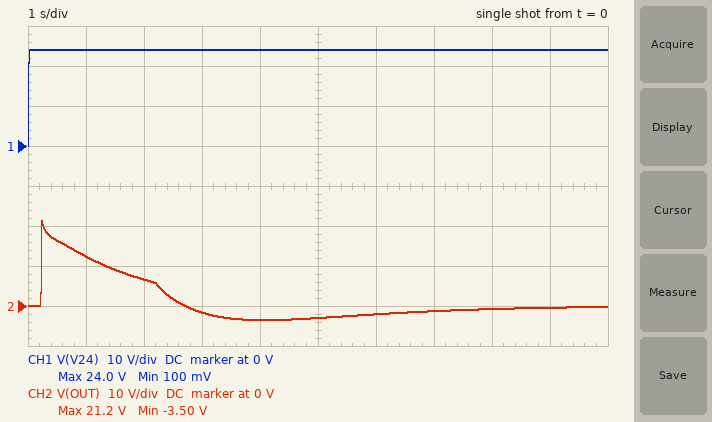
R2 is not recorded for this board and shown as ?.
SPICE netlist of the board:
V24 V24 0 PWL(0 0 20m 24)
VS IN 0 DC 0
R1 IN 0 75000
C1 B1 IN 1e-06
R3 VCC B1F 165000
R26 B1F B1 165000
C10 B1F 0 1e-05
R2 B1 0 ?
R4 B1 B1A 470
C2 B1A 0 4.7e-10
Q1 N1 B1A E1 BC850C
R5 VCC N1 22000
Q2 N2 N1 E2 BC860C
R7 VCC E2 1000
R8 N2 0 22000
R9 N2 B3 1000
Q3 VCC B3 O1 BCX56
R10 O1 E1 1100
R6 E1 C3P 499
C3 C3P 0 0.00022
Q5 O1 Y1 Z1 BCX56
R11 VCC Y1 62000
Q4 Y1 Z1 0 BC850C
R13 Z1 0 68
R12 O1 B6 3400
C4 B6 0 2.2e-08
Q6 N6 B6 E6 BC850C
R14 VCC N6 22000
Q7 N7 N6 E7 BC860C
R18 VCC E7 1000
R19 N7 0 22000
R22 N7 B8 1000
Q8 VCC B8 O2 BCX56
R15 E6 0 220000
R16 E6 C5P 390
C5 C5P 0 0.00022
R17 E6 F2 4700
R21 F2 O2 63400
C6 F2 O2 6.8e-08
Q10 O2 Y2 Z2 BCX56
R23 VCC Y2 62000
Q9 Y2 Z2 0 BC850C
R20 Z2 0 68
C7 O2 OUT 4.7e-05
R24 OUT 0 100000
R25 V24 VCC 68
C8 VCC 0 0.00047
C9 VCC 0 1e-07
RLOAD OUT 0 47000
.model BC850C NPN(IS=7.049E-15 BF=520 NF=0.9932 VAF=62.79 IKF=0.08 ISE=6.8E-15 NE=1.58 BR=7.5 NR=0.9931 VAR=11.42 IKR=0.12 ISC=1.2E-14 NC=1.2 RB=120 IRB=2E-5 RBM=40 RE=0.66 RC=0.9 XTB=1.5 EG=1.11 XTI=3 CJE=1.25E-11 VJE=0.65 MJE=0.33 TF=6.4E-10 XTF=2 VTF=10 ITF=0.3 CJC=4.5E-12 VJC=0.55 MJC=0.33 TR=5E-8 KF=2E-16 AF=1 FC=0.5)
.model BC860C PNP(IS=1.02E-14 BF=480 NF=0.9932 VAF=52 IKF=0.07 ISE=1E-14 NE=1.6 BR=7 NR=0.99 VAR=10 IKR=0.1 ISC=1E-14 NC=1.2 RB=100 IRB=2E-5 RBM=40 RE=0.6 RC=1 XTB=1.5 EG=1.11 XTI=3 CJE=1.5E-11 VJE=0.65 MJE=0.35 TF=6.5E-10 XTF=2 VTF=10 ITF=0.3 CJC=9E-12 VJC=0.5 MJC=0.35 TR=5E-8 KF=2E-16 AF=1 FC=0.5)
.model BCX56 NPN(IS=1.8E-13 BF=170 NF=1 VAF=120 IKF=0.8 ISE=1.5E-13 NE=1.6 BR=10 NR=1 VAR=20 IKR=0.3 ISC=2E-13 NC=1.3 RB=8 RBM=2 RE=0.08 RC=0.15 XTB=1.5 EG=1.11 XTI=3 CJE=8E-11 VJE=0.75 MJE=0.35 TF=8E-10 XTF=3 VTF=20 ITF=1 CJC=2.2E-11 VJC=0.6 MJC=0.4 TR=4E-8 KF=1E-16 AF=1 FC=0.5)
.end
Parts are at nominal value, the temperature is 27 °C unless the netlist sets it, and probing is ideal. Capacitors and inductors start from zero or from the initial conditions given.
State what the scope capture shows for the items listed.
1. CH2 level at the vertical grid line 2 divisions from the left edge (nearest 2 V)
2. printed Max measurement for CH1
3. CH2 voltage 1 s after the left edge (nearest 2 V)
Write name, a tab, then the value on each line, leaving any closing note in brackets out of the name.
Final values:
CH2 level at the vertical grid line 2 divisions from the left edge	6 V
printed Max measurement for CH1	24.0 V
CH2 voltage 1 s after the left edge	12 V
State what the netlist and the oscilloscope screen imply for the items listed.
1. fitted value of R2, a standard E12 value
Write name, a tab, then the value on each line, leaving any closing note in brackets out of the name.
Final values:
fitted value of R2, a standard E12 value	220 kΩ
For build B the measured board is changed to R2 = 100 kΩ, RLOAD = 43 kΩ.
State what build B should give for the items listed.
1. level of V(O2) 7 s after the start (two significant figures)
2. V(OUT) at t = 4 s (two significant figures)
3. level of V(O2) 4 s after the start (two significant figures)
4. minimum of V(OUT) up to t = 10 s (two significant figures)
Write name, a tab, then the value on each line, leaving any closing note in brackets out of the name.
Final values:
level of V(O2) 7 s after the start	2.9 V
V(OUT) at t = 4 s	-3.1 V
level of V(O2) 4 s after the start	4.0 V
minimum of V(OUT) up to t = 10 s	-3.8 V
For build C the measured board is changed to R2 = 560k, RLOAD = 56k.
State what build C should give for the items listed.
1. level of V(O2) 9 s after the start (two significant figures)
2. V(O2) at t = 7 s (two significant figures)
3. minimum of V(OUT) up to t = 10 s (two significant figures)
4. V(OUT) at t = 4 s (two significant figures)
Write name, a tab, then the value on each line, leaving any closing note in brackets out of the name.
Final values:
level of V(O2) 9 s after the start	13 V
V(O2) at t = 7 s	14 V
minimum of V(OUT) up to t = 10 s	-2.2 V
V(OUT) at t = 4 s	1.5 V
